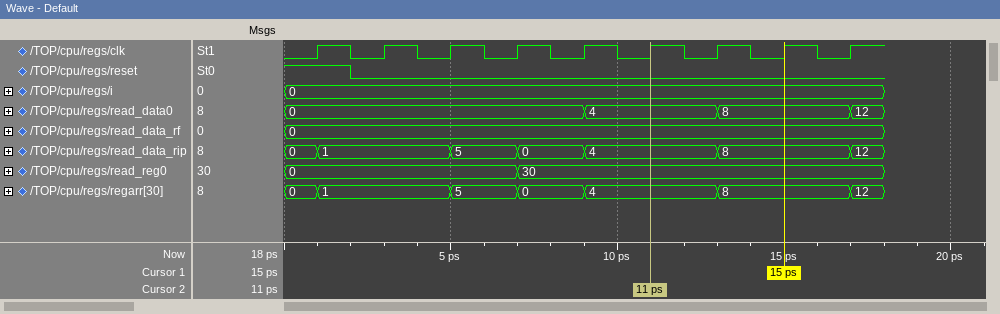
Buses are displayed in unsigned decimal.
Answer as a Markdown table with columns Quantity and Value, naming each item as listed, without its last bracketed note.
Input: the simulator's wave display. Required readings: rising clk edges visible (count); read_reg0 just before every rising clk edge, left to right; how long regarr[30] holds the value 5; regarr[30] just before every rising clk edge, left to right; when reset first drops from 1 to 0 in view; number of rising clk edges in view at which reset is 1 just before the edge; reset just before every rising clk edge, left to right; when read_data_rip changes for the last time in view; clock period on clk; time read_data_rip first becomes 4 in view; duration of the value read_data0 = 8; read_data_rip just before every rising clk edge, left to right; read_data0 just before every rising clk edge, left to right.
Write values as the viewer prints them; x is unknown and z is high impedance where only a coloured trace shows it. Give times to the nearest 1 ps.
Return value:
| Quantity | Value |
|---|---|
| rising clk edges visible | 9 |
| read_reg0 just before every rising clk edge, left to right | 0, 0, 0, 0, 30, 30, 30, 30, 30 |
| how long regarr[30] holds the value 5 | 2 ps |
| regarr[30] just before every rising clk edge, left to right | 0, 1, 1, 5, 0, 4, 4, 8, 8 |
| when reset first drops from 1 to 0 in view | 2 ps |
| number of rising clk edges in view at which reset is 1 just before the edge | 1 |
| reset just before every rising clk edge, left to right | 1 0 0 0 0 0 0 0 0 |
| when read_data_rip changes for the last time in view | 17 ps |
| clock period on clk | 2 ps |
| time read_data_rip first becomes 4 in view | 9 ps |
| duration of the value read_data0 = 8 | 4 ps |
| read_data_rip just before every rising clk edge, left to right | 0, 1, 1, 5, 0, 4, 4, 8, 8 |
| read_data0 just before every rising clk edge, left to right | 0, 0, 0, 0, 0, 4, 4, 8, 8 |
